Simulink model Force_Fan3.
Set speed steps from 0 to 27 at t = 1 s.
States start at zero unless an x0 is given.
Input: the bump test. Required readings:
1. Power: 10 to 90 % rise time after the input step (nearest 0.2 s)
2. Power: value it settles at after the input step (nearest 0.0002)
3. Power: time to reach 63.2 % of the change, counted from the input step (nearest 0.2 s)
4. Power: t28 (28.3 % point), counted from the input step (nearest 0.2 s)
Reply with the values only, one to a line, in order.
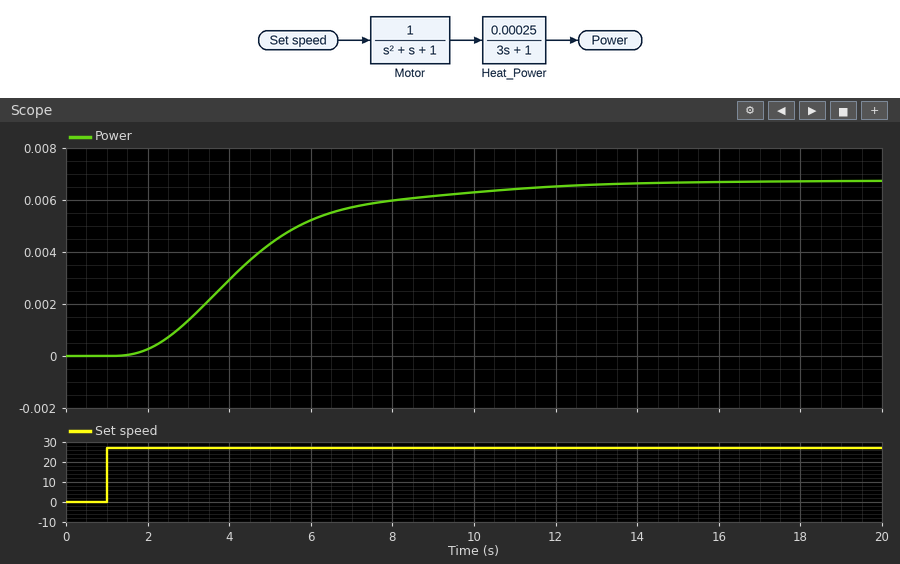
6.0 s
0.0068
4.0 s
2.4 s
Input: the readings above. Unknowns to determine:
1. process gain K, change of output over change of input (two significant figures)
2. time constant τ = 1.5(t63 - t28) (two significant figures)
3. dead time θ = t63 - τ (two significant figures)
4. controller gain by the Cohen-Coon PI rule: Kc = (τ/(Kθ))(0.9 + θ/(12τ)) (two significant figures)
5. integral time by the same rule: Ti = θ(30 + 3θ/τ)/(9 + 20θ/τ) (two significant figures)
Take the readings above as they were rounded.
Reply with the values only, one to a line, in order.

0.00025
2.4 s
1.6 s
5700
2.3 s
